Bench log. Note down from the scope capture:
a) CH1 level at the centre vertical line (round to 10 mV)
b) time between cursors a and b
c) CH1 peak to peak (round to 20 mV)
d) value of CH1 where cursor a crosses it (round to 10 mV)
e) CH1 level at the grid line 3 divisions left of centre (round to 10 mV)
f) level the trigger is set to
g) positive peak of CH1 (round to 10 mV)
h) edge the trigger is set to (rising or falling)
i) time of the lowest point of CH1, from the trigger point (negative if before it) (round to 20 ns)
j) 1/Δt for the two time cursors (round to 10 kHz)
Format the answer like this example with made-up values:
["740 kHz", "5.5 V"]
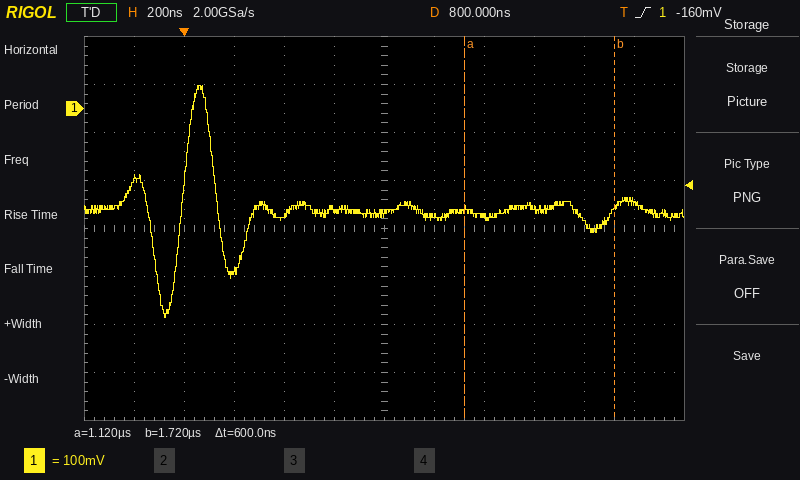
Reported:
["-220 mV", "600 ns", "480 mV", "-210 mV", "-340 mV", "-160 mV", "50 mV", "rising", "-80 ns", "1.67 MHz"]
